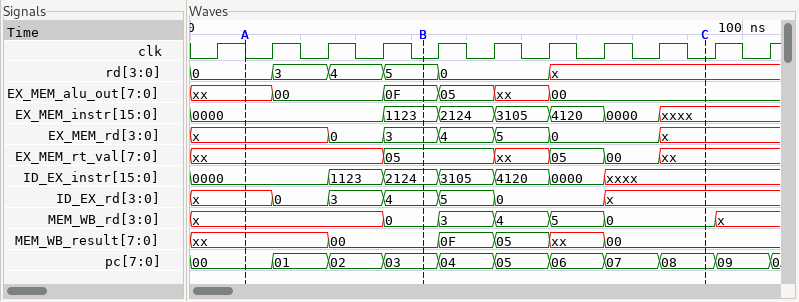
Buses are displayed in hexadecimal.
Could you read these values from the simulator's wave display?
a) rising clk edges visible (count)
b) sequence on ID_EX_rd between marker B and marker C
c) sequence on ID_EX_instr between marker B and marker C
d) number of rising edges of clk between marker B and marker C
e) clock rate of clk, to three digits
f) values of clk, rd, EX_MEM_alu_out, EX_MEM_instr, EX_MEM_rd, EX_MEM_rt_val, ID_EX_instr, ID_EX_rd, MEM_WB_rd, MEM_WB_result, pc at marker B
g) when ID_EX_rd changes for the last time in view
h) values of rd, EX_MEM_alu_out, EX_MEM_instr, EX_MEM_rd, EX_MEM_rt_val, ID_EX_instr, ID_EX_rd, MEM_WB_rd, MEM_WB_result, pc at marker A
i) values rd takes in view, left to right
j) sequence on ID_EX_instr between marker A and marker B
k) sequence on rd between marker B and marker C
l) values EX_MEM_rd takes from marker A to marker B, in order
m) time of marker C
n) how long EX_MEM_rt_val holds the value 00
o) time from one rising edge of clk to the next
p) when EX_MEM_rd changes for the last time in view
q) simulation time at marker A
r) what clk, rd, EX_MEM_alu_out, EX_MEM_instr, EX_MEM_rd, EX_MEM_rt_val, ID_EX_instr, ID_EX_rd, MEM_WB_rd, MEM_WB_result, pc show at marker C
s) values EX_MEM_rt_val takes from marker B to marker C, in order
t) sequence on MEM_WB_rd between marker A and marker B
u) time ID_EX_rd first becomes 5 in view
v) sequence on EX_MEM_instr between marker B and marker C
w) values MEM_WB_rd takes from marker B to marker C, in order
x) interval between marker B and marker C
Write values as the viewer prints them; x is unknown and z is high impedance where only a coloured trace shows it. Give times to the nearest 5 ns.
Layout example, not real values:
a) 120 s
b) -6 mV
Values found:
a) 11
b) 4, 5, 0, x
c) 2124, 3105, 4120, 0000, xxxx
d) 5
e) 100 MHz
f) clk=0, rd=5, EX_MEM_alu_out=0F, EX_MEM_instr=1123, EX_MEM_rd=3, EX_MEM_rt_val=05, ID_EX_instr=2124, ID_EX_rd=4, MEM_WB_rd=0, MEM_WB_result=00, pc=03
g) 75 ns
h) rd=0, EX_MEM_alu_out=xx, EX_MEM_instr=0000, EX_MEM_rd=x, EX_MEM_rt_val=xx, ID_EX_instr=0000, ID_EX_rd=x, MEM_WB_rd=x, MEM_WB_result=xx, pc=00
i) 0, 3, 4, 5, 0, x
j) 0000, 1123, 2124
k) 5, 0, x
l) x, 0, 3
m) 95 ns
n) 10 ns
o) 10 ns
p) 85 ns
q) 10 ns
r) clk=0, rd=x, EX_MEM_alu_out=00, EX_MEM_instr=xxxx, EX_MEM_rd=x, EX_MEM_rt_val=xx, ID_EX_instr=xxxx, ID_EX_rd=x, MEM_WB_rd=0, MEM_WB_result=00, pc=08
s) 05, xx, 05, 00, xx
t) x, 0
u) 45 ns
v) 1123, 2124, 3105, 4120, 0000, xxxx
w) 0, 3, 4, 5, 0
x) 50 ns
